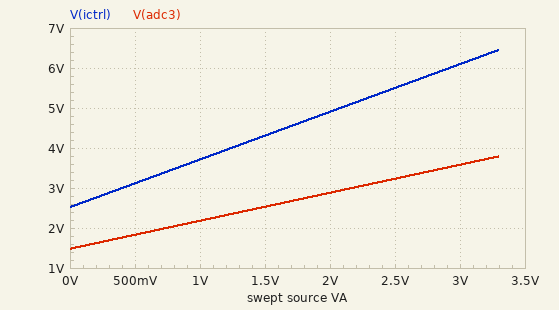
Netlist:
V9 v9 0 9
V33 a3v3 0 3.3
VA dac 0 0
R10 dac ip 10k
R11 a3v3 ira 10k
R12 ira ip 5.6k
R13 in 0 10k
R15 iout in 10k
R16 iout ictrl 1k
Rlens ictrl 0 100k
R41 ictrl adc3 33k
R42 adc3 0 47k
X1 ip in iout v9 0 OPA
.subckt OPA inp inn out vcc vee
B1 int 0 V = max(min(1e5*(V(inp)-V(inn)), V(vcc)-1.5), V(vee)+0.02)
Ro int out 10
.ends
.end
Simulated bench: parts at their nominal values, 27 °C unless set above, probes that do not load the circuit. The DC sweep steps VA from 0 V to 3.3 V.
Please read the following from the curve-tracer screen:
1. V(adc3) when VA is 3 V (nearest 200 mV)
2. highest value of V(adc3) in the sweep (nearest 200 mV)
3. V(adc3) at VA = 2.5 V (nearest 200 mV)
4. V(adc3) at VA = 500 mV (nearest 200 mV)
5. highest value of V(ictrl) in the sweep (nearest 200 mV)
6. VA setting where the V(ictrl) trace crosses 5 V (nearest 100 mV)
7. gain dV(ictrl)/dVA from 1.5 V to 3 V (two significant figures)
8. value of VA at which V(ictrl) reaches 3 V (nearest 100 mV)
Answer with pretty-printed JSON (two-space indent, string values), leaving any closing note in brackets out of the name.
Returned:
{
  "V(adc3) when VA is 3 V": "3.6 V",
  "highest value of V(adc3) in the sweep": "3.8 V",
  "V(adc3) at VA = 2.5 V": "3.2 V",
  "V(adc3) at VA = 500 mV": "1.8 V",
  "highest value of V(ictrl) in the sweep": "6.4 V",
  "VA setting where the V(ictrl) trace crosses 5 V": "2.1 V",
  "gain dV(ictrl)/dVA from 1.5 V to 3 V": "1.2 V/V",
  "value of VA at which V(ictrl) reaches 3 V": "400 mV"
}
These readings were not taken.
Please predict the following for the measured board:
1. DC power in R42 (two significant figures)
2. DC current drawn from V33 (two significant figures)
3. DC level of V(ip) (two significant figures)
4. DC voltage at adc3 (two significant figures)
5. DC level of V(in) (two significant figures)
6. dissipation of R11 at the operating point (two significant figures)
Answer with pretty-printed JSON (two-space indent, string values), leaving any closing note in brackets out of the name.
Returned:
{
  "DC power in R42": "47 µW",
  "DC current drawn from V33": "130 µA",
  "DC level of V(ip)": "1.3 V",
  "DC voltage at adc3": "1.5 V",
  "DC level of V(in)": "1.3 V",
  "dissipation of R11 at the operating point": "170 µW"
}
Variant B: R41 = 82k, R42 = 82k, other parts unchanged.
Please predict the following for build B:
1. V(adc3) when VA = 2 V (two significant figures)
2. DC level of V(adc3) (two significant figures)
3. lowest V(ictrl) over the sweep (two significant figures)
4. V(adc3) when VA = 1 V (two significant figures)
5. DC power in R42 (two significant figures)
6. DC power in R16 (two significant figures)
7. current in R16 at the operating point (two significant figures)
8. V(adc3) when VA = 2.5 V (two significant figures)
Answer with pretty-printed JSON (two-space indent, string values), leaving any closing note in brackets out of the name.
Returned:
{
  "V(adc3) when VA = 2 V": "2.5 V",
  "DC level of V(adc3)": "1.3 V",
  "lowest V(ictrl) over the sweep": "2.5 V",
  "V(adc3) when VA = 1 V": "1.9 V",
  "DC power in R42": "20 µW",
  "DC power in R16": "1.7 µW",
  "current in R16 at the operating point": "41 µA",
  "V(adc3) when VA = 2.5 V": "2.8 V"
}
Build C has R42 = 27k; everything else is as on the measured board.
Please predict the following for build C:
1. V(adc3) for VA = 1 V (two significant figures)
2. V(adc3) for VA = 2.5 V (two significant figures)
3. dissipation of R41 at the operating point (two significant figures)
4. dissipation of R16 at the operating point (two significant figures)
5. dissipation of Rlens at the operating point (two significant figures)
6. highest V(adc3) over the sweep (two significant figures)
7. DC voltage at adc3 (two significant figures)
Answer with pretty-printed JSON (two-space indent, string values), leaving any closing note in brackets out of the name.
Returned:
{
  "V(adc3) for VA = 1 V": "1.7 V",
  "V(adc3) for VA = 2.5 V": "2.5 V",
  "dissipation of R41 at the operating point": "58 µW",
  "dissipation of R16 at the operating point": "4.5 µW",
  "dissipation of Rlens at the operating point": "63 µW",
  "highest V(adc3) over the sweep": "2.9 V",
  "DC voltage at adc3": "1.1 V"
}
